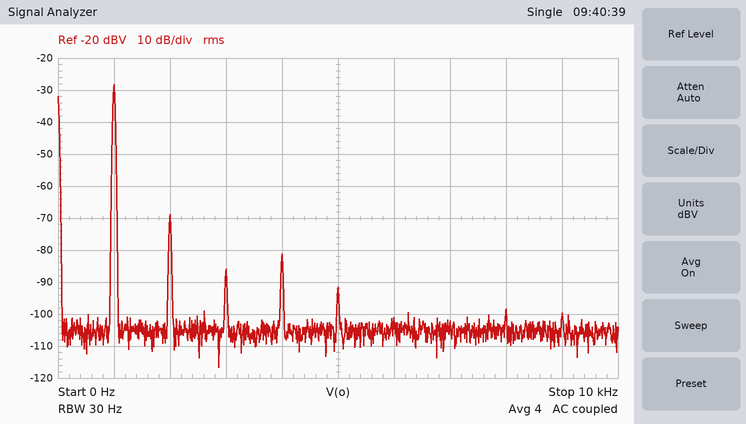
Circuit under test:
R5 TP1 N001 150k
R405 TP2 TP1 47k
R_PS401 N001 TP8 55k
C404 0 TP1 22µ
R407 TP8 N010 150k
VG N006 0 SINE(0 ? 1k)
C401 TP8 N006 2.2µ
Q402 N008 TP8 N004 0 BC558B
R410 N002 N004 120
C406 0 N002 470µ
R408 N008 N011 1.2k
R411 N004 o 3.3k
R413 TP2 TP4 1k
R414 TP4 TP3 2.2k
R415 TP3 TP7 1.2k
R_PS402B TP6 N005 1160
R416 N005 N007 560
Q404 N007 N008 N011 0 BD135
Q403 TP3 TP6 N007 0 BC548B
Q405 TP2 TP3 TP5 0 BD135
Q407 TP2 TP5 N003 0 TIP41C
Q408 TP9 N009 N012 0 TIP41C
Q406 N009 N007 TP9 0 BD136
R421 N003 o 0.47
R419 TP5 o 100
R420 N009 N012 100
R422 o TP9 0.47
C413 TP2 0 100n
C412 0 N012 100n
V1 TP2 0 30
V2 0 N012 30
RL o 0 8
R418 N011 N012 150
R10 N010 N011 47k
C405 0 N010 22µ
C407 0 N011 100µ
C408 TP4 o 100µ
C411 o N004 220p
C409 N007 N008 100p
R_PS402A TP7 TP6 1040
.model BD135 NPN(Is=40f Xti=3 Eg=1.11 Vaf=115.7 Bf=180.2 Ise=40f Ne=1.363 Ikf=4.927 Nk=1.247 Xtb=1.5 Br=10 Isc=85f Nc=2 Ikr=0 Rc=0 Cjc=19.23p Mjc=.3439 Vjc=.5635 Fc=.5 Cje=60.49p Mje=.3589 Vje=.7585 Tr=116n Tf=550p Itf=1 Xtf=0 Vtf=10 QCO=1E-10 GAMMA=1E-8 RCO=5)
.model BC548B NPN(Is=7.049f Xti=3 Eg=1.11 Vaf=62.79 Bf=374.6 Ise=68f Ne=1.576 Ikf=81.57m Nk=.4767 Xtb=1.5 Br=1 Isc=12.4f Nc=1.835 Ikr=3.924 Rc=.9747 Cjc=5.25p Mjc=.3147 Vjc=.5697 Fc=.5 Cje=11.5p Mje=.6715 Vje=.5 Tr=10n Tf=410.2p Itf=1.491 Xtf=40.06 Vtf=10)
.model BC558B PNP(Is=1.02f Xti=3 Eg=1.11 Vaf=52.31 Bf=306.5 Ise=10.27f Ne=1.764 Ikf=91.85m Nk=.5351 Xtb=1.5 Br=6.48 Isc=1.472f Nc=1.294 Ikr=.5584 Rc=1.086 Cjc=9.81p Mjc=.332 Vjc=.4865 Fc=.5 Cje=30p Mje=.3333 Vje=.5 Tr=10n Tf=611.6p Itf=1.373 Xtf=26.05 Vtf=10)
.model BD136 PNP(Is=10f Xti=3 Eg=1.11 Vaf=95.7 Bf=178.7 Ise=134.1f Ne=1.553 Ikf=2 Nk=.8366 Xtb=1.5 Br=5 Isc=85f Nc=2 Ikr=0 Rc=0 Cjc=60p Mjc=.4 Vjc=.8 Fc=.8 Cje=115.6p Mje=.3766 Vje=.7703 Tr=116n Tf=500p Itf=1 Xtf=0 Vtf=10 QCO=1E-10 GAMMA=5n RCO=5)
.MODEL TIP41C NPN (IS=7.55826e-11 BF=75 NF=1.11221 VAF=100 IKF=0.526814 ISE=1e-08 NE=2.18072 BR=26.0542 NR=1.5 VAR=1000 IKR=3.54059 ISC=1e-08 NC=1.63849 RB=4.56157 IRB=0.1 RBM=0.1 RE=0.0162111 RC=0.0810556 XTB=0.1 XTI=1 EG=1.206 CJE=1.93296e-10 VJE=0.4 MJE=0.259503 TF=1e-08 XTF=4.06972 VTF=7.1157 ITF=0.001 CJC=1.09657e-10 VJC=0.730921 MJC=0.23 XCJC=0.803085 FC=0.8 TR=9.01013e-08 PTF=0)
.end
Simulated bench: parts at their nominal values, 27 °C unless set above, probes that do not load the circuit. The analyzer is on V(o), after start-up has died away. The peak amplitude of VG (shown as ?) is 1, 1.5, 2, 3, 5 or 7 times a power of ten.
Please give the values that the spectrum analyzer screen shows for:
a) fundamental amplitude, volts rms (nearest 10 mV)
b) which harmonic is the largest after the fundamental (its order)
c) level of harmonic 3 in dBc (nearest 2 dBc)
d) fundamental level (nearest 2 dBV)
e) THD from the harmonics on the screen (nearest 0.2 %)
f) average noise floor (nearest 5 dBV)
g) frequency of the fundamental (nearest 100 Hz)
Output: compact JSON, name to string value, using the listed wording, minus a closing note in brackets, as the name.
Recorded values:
{"fundamental amplitude, volts rms": "40 mV", "which harmonic is the largest after the fundamental": "2", "level of harmonic 3 in dBc": "-58 dBc", "fundamental level": "-28 dBV", "THD from the harmonics on the screen": "1.0 %", "average noise floor": "-105 dBV", "frequency of the fundamental": "1.0 kHz"}
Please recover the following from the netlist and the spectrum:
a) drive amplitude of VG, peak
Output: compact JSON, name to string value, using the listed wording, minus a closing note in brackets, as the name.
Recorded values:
{"drive amplitude of VG, peak": "2 mV"}
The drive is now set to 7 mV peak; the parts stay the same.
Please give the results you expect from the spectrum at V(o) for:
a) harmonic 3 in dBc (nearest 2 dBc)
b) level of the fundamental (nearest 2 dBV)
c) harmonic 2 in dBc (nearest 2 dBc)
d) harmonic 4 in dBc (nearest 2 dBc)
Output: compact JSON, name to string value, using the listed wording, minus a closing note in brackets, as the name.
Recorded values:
{"harmonic 3 in dBc": "-50 dBc", "level of the fundamental": "-18 dBV", "harmonic 2 in dBc": "-52 dBc", "harmonic 4 in dBc": "-56 dBc"}
